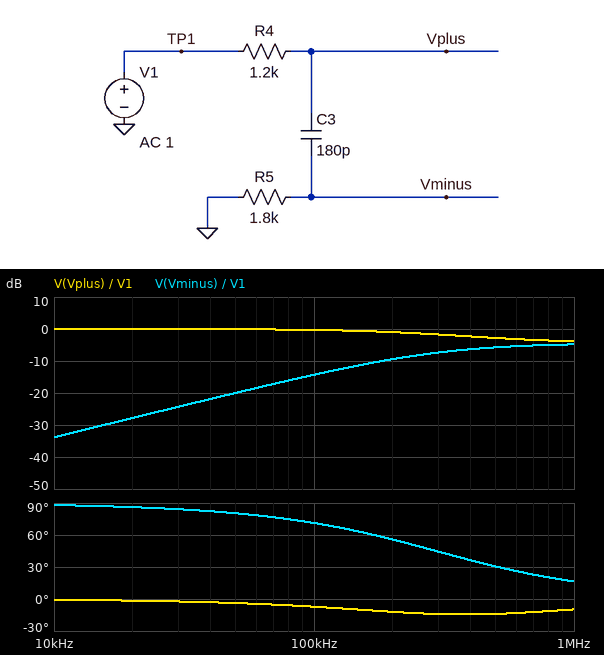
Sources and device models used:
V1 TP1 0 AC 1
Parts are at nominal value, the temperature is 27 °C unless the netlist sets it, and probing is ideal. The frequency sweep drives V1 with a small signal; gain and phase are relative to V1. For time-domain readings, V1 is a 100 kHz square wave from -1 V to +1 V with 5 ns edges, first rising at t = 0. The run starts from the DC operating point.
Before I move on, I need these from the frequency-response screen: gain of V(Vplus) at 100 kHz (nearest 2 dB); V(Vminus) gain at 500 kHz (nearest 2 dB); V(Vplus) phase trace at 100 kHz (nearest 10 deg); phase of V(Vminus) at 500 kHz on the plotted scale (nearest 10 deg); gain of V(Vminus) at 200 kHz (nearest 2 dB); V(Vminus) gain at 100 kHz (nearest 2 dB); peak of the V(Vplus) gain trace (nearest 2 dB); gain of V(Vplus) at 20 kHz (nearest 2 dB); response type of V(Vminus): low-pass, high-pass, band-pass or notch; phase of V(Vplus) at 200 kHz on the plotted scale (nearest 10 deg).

0 dB
-6 dB
-10 deg
30 deg
-10 dB
-14 dB
0 dB
0 dB
high-pass
-10 deg
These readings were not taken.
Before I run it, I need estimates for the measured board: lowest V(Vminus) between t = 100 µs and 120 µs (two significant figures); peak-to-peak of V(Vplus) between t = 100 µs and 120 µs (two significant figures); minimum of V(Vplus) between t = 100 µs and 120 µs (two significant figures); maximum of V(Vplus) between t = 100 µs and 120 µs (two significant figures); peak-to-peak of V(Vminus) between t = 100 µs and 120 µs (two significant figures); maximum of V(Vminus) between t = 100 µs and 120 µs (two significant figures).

-1.2 V
2.0 V
-1.0 V
1.0 V
2.4 V
1.2 V
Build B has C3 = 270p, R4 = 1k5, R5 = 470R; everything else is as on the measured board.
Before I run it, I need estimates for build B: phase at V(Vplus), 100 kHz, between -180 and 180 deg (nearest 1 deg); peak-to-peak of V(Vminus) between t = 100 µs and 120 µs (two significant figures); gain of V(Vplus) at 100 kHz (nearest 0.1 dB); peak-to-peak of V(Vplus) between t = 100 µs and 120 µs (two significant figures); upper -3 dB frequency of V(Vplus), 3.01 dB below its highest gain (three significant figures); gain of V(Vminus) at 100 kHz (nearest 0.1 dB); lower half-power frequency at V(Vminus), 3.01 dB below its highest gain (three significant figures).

-14 deg
950 mV
-0.4 dB
2.0 V
318 kHz
-22.4 dB
299 kHz
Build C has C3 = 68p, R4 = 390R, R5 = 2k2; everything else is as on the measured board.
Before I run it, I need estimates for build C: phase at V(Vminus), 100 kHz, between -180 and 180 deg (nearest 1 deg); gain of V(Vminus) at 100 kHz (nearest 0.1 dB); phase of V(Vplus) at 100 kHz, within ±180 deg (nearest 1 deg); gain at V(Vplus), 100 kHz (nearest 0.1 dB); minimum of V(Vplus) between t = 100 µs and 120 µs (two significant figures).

84 deg
-20.6 dB
-1 deg
0 dB
-1.0 V
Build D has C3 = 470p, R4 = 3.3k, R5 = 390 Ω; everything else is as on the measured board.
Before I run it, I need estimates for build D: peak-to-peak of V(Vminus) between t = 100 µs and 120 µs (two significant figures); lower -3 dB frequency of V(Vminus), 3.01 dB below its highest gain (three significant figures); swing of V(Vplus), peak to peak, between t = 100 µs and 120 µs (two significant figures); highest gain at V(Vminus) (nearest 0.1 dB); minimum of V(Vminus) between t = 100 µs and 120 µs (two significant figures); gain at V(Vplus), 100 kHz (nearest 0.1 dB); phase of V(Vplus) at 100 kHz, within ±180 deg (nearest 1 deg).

400 mV
91.8 kHz
1.8 V
-19.5 dB
-200 mV
-3.3 dB
-41 deg
